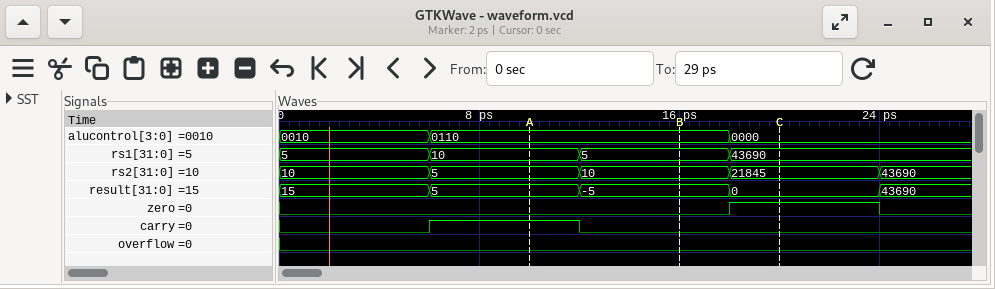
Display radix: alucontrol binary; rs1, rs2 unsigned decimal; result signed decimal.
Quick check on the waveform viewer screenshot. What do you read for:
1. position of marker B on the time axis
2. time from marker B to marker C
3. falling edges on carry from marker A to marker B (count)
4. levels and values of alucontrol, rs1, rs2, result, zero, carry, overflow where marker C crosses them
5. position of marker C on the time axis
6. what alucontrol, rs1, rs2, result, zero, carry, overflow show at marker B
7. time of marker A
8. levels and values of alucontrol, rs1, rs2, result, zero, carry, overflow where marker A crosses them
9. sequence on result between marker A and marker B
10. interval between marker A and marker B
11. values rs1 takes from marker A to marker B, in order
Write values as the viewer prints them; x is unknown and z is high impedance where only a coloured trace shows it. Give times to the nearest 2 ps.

16 ps
4 ps
1
alucontrol=0000, rs1=43690, rs2=21845, result=0, zero=1, carry=0, overflow=0
20 ps
alucontrol=0110, rs1=5, rs2=10, result=-5, zero=0, carry=0, overflow=0
10 ps
alucontrol=0110, rs1=10, rs2=5, result=5, zero=0, carry=1, overflow=0
5, -5
6 ps
10, 5
